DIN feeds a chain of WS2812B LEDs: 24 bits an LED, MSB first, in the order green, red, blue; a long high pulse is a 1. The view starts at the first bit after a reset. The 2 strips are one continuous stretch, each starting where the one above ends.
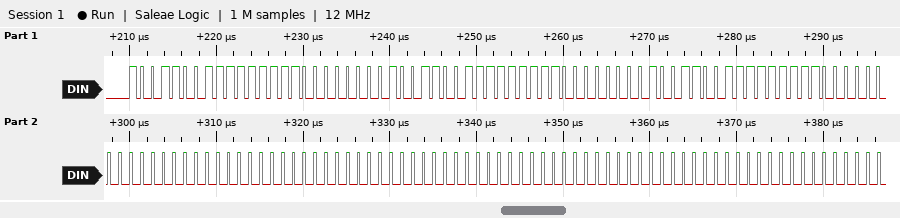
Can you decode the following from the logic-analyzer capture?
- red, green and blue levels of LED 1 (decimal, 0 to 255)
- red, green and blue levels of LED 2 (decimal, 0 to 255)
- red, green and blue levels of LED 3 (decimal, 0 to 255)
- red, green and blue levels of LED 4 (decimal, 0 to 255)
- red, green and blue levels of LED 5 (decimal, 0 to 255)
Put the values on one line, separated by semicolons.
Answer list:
255, 153, 0; 255, 153, 0; 255, 153, 0; 0, 0, 0; 0, 0, 0
